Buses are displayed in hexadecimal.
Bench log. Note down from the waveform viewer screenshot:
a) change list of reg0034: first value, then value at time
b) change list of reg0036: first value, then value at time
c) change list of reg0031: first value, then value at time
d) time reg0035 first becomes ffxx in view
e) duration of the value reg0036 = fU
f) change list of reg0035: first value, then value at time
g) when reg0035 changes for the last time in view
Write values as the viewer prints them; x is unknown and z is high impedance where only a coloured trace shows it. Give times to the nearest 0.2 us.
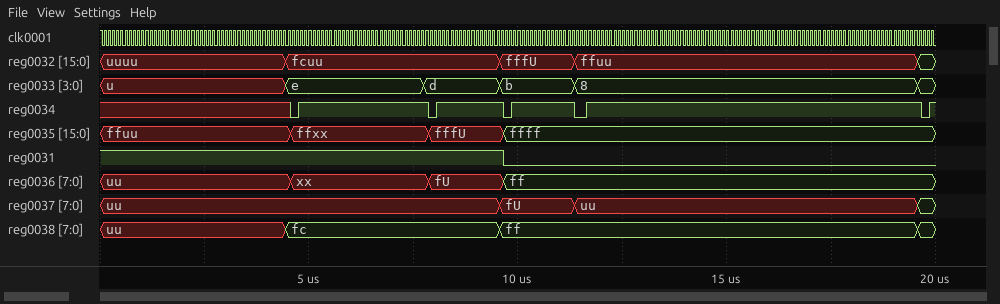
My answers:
x, 0 at 4.6 us, 1 at 4.8 us, 0 at 7.8 us, 1 at 8 us, 0 at 9.6 us, 1 at 9.8 us, 0 at 11.4 us, 1 at 11.6 us, 0 at 19.6 us, 1 at 19.8 us
uu, xx at 4.6 us, fU at 7.8 us, ff at 9.6 us
1, 0 at 9.6 us
4.6 us
1.8 us
ffuu, ffxx at 4.6 us, fffU at 7.8 us, ffff at 9.6 us
9.6 us
